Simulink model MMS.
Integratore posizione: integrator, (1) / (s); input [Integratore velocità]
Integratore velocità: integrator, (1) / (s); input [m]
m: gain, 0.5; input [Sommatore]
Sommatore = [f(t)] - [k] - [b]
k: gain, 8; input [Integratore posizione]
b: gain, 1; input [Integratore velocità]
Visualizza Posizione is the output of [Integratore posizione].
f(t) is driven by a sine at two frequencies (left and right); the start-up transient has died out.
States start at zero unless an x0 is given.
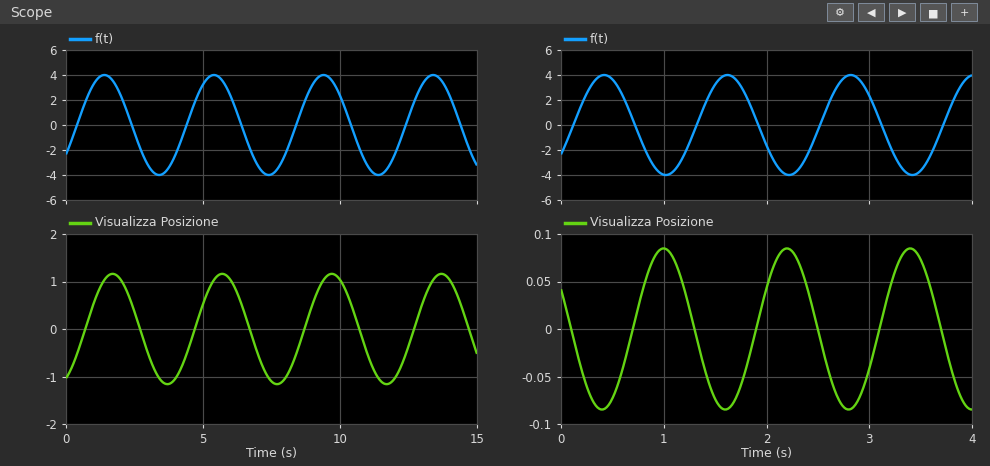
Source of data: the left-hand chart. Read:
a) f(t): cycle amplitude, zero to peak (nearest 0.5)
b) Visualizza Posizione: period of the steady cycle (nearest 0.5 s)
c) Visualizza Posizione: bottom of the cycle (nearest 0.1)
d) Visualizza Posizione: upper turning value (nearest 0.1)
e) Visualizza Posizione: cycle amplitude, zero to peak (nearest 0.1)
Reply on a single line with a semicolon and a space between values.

4.0; 4.0 s; -1.2; 1.2; 1.2
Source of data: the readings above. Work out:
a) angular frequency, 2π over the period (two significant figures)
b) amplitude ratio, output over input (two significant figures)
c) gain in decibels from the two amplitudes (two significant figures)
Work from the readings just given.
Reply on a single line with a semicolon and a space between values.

1.6 rad/s; 0.30; -10 dB
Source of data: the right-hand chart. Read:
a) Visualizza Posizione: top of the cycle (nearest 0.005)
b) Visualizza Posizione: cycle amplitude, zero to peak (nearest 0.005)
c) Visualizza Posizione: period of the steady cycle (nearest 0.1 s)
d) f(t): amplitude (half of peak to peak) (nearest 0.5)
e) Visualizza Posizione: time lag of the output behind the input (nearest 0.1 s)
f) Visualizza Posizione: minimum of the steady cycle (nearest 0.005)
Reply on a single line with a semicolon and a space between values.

0.085; 0.085; 1.2 s; 4.0; 0.6 s; -0.085
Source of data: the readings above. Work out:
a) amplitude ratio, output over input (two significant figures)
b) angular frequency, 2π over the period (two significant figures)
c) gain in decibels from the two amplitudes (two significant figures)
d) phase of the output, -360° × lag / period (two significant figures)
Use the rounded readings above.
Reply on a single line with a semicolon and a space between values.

0.021; 5.2 rad/s; -33 dB; -180°
